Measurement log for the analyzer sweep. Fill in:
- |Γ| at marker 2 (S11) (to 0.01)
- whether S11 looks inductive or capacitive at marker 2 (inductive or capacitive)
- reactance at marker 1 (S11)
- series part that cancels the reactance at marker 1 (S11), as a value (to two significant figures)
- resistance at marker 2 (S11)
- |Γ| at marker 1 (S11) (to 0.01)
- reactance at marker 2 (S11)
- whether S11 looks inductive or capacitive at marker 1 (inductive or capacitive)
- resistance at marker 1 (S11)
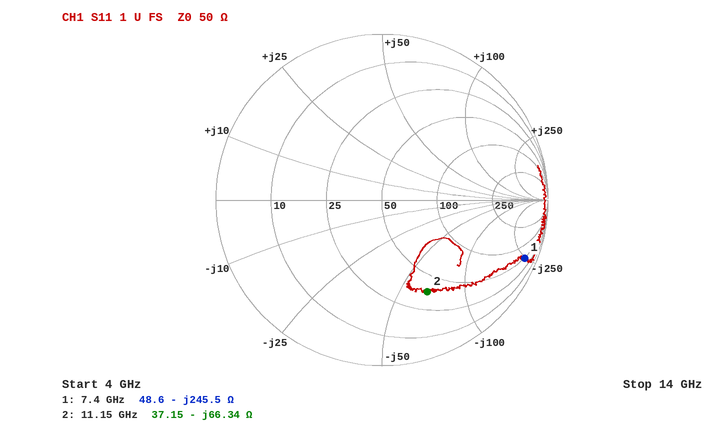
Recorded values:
0.62
capacitive
-245.5 Ω
5.3 nH
37.15 Ω
0.93
-66.34 Ω
capacitive
48.6 Ω
